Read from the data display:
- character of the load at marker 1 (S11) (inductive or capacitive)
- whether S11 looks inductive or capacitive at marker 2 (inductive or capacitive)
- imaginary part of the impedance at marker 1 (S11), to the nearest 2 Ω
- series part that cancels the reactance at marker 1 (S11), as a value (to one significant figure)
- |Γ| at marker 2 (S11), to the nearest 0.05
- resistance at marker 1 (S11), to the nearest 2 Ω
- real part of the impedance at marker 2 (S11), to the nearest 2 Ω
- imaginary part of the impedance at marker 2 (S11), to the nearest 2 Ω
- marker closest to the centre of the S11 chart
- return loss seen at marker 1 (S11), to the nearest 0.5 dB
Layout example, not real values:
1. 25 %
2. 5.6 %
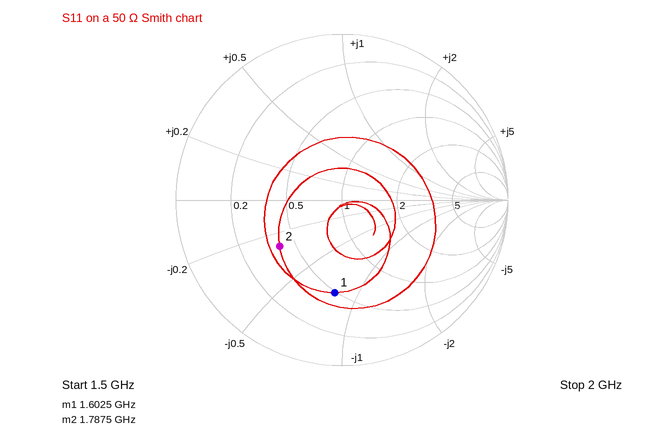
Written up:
1. capacitive
2. capacitive
3. -40 Ω
4. 4 nH
5. 0.45
6. 24 Ω
7. 20 Ω
8. -14 Ω
9. marker 2
10. 5.0 dB
